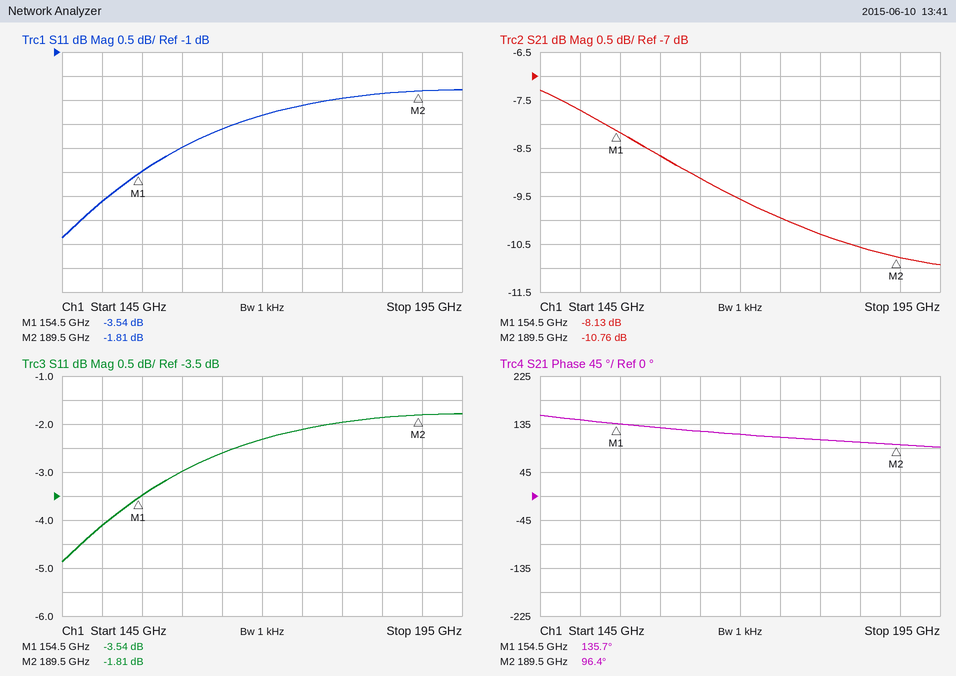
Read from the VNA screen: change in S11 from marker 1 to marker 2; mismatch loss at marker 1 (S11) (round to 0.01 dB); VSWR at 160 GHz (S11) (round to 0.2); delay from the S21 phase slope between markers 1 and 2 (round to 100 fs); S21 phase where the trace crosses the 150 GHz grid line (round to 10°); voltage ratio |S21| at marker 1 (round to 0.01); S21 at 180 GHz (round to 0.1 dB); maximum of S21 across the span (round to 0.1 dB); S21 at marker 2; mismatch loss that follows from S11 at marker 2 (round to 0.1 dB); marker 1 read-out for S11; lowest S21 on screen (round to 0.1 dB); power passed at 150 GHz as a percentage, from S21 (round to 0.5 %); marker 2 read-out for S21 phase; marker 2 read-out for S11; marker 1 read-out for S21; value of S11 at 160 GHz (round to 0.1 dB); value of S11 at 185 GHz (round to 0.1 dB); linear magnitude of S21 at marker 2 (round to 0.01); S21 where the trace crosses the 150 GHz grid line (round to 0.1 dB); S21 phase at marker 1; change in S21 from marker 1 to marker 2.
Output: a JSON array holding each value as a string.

["1.73 dB", "2.54 dB", "5.8", "3.1 ps", "140°", "0.39", "-10.3 dB", "-7.3 dB", "-10.76 dB", "4.7 dB", "-3.54 dB", "-10.9 dB", "17.0 %", "96.4°", "-1.81 dB", "-8.13 dB", "-3.0 dB", "-1.9 dB", "0.29", "-7.7 dB", "135.7°", "-2.63 dB"]
